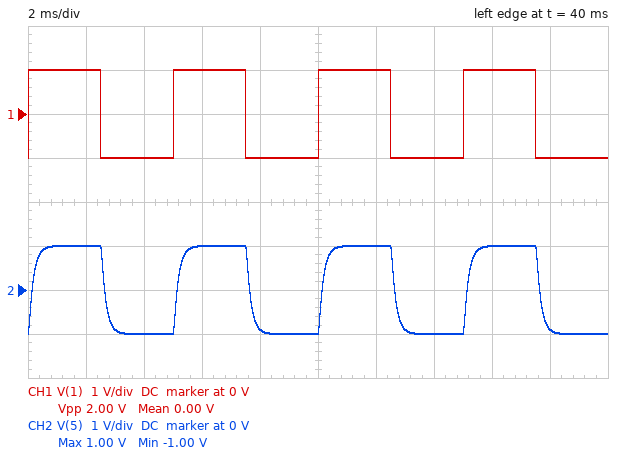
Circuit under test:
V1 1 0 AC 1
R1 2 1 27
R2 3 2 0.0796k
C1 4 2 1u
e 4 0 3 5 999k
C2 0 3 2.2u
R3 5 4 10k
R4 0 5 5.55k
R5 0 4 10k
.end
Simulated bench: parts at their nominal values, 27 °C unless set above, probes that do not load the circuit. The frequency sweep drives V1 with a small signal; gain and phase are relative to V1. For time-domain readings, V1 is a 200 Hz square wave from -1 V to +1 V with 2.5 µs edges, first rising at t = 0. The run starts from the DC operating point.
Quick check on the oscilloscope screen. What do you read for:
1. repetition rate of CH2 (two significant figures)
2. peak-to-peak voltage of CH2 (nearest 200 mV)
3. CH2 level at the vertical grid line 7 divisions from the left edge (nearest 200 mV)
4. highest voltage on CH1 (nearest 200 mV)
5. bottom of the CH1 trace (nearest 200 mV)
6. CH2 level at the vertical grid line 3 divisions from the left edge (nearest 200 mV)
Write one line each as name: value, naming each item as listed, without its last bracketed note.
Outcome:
repetition rate of CH2: 200 Hz
peak-to-peak voltage of CH2: 2.0 V
CH2 level at the vertical grid line 7 divisions from the left edge: -1.0 V
highest voltage on CH1: 1.0 V
bottom of the CH1 trace: -1.0 V
CH2 level at the vertical grid line 3 divisions from the left edge: 1.0 V
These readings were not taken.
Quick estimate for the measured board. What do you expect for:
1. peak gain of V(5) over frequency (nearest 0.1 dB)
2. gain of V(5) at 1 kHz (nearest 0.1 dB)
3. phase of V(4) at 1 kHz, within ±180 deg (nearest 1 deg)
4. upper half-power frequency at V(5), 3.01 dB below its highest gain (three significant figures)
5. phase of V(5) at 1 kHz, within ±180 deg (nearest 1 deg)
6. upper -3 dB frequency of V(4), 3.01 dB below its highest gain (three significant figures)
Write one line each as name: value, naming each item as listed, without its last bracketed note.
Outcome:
peak gain of V(5) over frequency: 0 dB
gain of V(5) at 1 kHz: -3.1 dB
phase of V(4) at 1 kHz, within ±180 deg: -55 deg
upper half-power frequency at V(5), 3.01 dB below its highest gain: 988 Hz
phase of V(5) at 1 kHz, within ±180 deg: -55 deg
upper -3 dB frequency of V(4), 3.01 dB below its highest gain: 988 Hz
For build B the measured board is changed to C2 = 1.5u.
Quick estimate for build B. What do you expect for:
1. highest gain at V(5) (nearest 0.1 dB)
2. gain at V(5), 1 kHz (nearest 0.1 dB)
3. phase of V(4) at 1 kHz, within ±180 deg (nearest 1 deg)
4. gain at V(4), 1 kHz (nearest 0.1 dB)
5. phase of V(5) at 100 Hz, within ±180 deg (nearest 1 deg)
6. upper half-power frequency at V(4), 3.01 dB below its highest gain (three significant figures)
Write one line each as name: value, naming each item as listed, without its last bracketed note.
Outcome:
highest gain at V(5): 0 dB
gain at V(5), 1 kHz: -1.0 dB
phase of V(4) at 1 kHz, within ±180 deg: -39 deg
gain at V(4), 1 kHz: 8.0 dB
phase of V(5) at 100 Hz, within ±180 deg: -4 deg
upper half-power frequency at V(4), 3.01 dB below its highest gain: 1.86 kHz
